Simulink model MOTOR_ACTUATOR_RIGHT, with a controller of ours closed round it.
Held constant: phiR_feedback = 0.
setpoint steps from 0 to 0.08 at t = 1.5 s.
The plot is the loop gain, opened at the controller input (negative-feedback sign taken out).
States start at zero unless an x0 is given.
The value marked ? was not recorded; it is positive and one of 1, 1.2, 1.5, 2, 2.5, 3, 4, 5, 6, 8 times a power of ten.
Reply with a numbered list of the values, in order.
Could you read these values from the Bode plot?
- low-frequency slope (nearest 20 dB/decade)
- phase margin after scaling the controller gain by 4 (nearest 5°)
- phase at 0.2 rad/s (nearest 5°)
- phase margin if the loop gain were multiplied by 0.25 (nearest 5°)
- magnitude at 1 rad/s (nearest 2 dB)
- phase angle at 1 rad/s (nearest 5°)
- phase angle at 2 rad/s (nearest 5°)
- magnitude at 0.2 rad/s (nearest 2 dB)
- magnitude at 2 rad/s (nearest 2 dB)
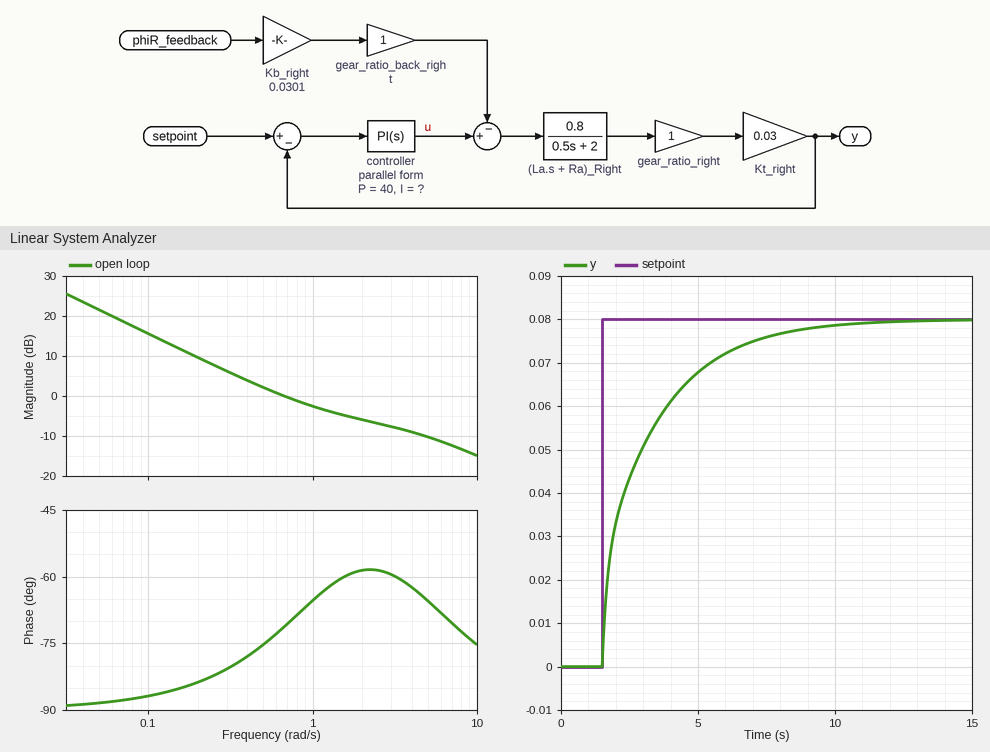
1. -20 dB/decade
2. 110°
3. -85°
4. 95°
5. -2 dB
6. -65°
7. -60°
8. 10 dB
9. -6 dB
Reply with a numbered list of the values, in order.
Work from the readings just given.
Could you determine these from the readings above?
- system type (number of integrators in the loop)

1. 1
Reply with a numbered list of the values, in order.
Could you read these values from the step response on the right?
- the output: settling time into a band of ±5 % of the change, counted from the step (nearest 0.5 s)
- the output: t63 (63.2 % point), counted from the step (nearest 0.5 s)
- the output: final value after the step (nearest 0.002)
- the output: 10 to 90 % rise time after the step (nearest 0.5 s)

1. 6.0 s
2. 1.5 s
3. 0.080
4. 4.5 s
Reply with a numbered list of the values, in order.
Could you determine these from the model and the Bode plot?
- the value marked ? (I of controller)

1. 50
